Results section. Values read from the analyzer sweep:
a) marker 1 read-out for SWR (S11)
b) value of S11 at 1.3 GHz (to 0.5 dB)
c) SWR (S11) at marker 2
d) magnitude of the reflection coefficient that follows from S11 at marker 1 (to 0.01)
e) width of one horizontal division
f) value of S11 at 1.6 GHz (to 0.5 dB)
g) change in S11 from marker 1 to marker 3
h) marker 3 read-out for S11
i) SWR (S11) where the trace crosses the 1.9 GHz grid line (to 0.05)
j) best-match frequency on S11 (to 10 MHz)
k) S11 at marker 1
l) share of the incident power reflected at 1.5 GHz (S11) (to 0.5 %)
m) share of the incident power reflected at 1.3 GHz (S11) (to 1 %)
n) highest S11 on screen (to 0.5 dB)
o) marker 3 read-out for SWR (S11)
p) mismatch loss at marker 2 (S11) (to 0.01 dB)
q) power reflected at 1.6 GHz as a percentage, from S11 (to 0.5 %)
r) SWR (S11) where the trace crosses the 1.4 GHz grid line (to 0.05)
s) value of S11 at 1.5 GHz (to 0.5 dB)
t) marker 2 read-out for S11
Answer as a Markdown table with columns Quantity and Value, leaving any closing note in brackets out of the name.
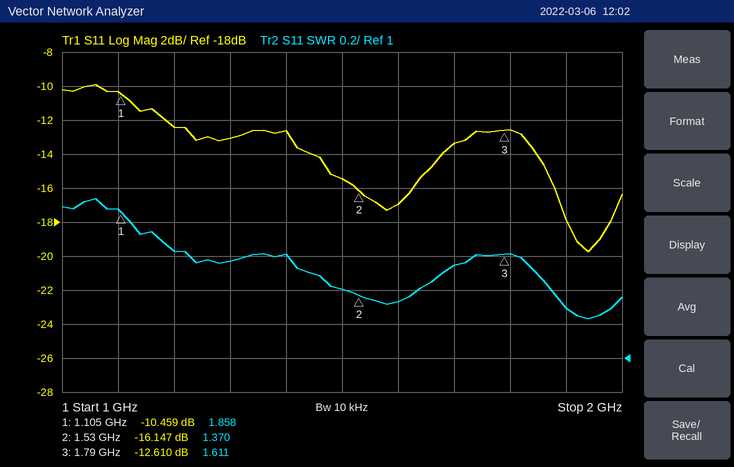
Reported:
| Quantity | Value |
|---|---|
| marker 1 read-out for SWR | 1.858 |
| value of S11 at 1.3 GHz | -13.0 dB |
| SWR (S11) at marker 2 | 1.370 |
| magnitude of the reflection coefficient that follows from S11 at marker 1 | 0.30 |
| width of one horizontal division | 100 MHz |
| value of S11 at 1.6 GHz | -17.0 dB |
| change in S11 from marker 1 to marker 3 | -2.151 dB |
| marker 3 read-out for S11 | -12.610 dB |
| SWR (S11) where the trace crosses the 1.9 GHz grid line | 1.30 |
| best-match frequency on S11 | 1.94 GHz |
| S11 at marker 1 | -10.459 dB |
| share of the incident power reflected at 1.5 GHz (S11) | 3.0 % |
| share of the incident power reflected at 1.3 GHz (S11) | 5 % |
| highest S11 on screen | -10.0 dB |
| marker 3 read-out for SWR | 1.611 |
| mismatch loss at marker 2 (S11) | 0.11 dB |
| power reflected at 1.6 GHz as a percentage, from S11 | 2.0 % |
| SWR (S11) where the trace crosses the 1.4 GHz grid line | 1.60 |
| value of S11 at 1.5 GHz | -15.5 dB |
| marker 2 read-out for S11 | -16.147 dB |
